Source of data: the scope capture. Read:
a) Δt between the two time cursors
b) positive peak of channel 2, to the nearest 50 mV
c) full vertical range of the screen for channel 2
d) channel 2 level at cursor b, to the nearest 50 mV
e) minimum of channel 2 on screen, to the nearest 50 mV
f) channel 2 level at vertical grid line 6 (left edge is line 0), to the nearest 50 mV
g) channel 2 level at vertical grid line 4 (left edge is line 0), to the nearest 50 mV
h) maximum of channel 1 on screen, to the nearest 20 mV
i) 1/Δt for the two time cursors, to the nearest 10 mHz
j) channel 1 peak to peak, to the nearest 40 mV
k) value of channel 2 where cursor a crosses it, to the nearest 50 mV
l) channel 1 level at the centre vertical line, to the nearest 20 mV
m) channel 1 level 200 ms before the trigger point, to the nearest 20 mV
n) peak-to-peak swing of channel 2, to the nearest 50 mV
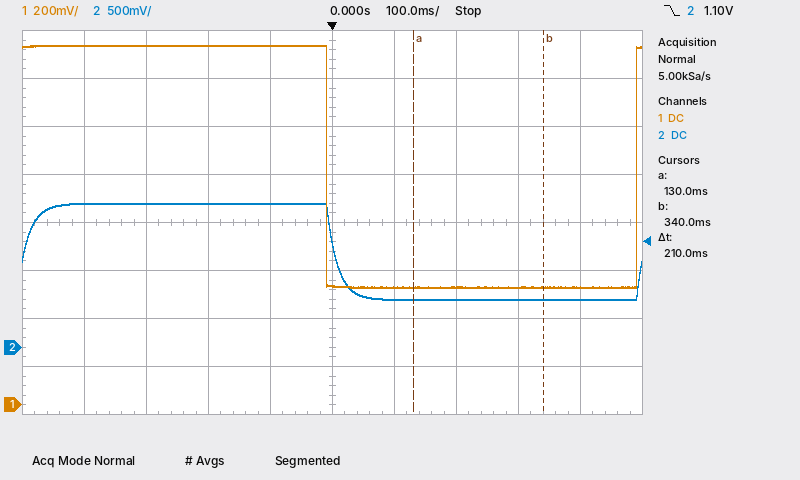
210 ms
1.50 V
4 V
500 mV
500 mV
500 mV
1.50 V
1.50 V
4.76 Hz
1.00 V
500 mV
500 mV
1.50 V
1.00 V
